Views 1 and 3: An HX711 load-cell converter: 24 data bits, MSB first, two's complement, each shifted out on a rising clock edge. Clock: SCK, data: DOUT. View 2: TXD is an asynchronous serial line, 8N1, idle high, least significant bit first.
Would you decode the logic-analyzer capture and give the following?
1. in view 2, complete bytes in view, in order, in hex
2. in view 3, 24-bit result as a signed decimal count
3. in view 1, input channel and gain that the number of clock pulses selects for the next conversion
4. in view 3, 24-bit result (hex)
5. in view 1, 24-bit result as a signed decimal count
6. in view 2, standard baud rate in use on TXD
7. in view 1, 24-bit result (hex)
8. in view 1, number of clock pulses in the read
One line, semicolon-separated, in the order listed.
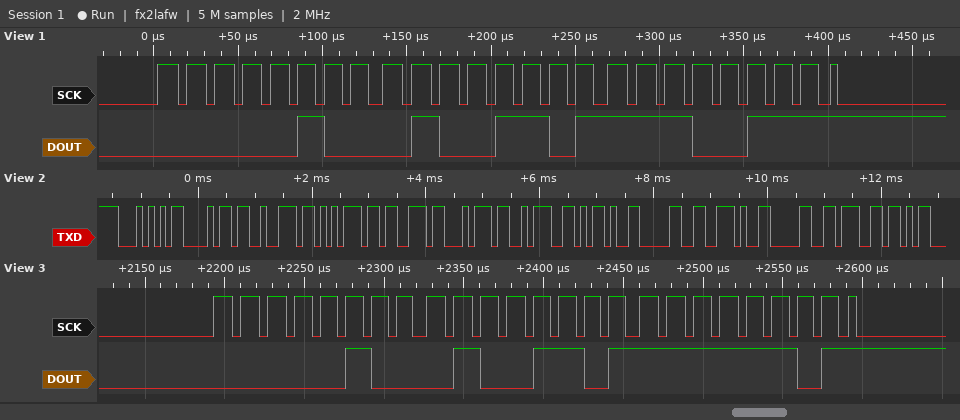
0x54 0x68 0x72 0x75 0x73 0x74 0x3A 0x2D 0x30 0x2E 0x30 0x67; 282109; channel A, gain 128; 0x044DFD; 282087; 9600 baud; 0x044DE7; 25
